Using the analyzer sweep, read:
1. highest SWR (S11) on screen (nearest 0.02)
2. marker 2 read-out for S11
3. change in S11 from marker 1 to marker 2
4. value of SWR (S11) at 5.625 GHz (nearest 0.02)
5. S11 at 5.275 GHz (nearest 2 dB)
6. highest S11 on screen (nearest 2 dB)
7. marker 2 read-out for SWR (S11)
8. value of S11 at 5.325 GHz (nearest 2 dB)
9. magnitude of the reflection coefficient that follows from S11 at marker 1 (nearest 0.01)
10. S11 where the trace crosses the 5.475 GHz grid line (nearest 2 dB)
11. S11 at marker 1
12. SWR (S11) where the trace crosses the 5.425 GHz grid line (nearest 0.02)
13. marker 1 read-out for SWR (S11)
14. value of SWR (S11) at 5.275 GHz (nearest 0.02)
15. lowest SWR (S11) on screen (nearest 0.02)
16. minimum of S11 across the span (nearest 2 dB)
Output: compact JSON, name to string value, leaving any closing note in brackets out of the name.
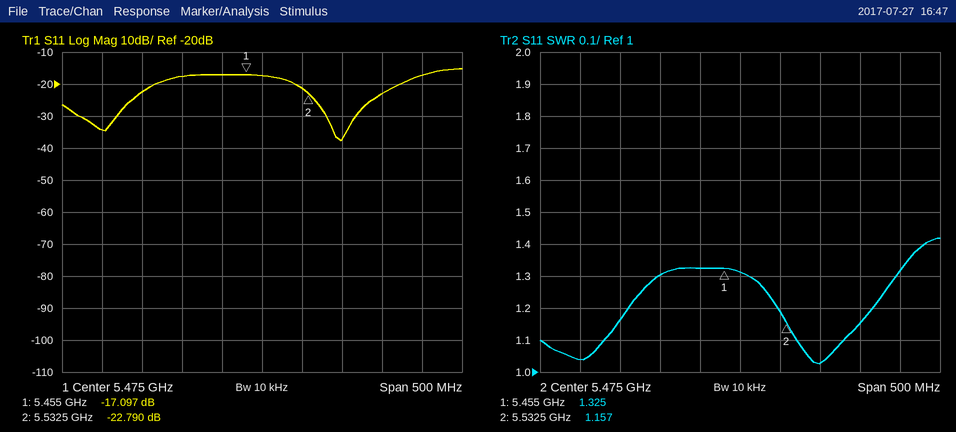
{"highest SWR (S11) on screen": "1.42", "marker 2 read-out for S11": "-22.790 dB", "change in S11 from marker 1 to marker 2": "-5.693 dB", "value of SWR (S11) at 5.625 GHz": "1.16", "S11 at 5.275 GHz": "-34 dB", "highest S11 on screen": "-16 dB", "marker 2 read-out for SWR": "1.157", "value of S11 at 5.325 GHz": "-22 dB", "magnitude of the reflection coefficient that follows from S11 at marker 1": "0.14", "S11 where the trace crosses the 5.475 GHz grid line": "-18 dB", "S11 at marker 1": "-17.097 dB", "SWR (S11) where the trace crosses the 5.425 GHz grid line": "1.32", "marker 1 read-out for SWR": "1.325", "value of SWR (S11) at 5.275 GHz": "1.04", "lowest SWR (S11) on screen": "1.02", "minimum of S11 across the span": "-38 dB"}
